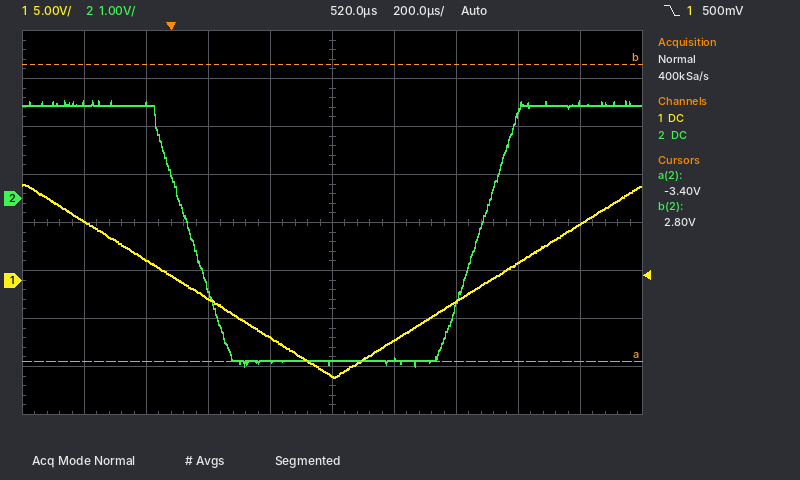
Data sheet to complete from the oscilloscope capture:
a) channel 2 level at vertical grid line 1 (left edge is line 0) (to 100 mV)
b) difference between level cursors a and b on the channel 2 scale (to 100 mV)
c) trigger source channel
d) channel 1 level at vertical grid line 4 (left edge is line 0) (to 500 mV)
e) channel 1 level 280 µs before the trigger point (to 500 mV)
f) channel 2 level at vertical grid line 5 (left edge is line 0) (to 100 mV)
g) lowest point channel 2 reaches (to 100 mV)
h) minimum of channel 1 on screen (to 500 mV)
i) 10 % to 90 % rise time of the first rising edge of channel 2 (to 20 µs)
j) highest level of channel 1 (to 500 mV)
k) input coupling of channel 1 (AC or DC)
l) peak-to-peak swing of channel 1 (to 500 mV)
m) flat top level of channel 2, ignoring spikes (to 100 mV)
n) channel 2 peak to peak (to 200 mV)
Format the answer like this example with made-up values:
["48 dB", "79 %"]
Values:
["2.0 V", "6.2 V", "channel 1", "-6.0 V", "6.0 V", "-3.4 V", "-3.5 V", "-10.0 V", "220 µs", "10.0 V", "DC", "20.0 V", "1.9 V", "5.6 V"]
